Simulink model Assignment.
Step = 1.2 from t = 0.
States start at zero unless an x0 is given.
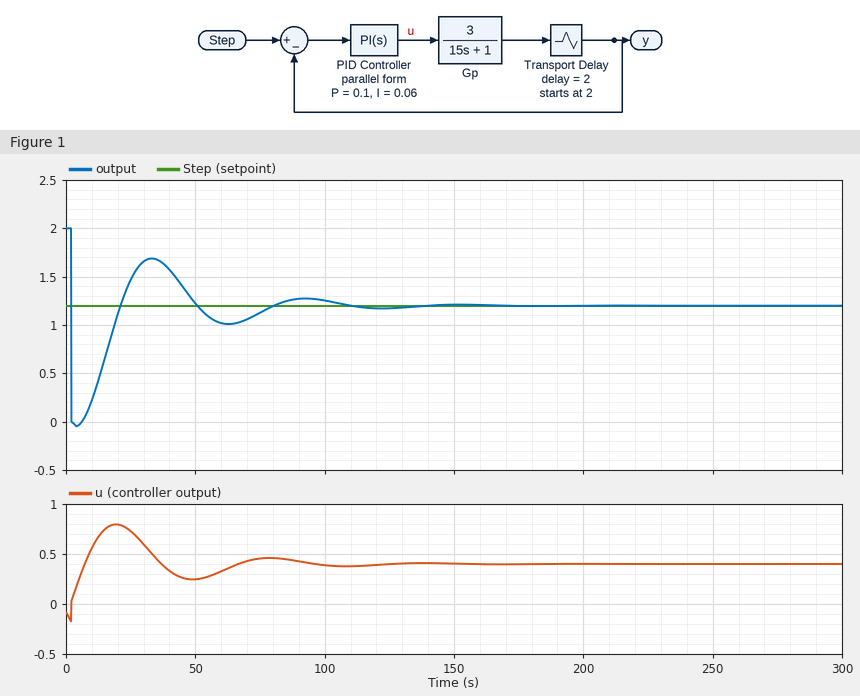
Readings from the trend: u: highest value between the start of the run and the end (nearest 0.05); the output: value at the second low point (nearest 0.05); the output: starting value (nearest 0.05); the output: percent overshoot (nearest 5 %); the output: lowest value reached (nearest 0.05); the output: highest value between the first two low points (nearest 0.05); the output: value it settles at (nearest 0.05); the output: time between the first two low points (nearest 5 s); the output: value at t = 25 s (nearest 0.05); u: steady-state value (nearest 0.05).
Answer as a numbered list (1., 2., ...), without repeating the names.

1. 0.80
2. 1.00
3. 2.00
4. 155 %
5. -0.05
6. 1.70
7. 1.20
8. 60 s
9. 1.45
10. 0.40
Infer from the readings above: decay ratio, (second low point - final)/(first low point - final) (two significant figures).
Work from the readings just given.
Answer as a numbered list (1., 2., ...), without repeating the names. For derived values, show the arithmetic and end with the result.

1. (1 - 1.2) / (-0.05 - 1.2) = 0.16
